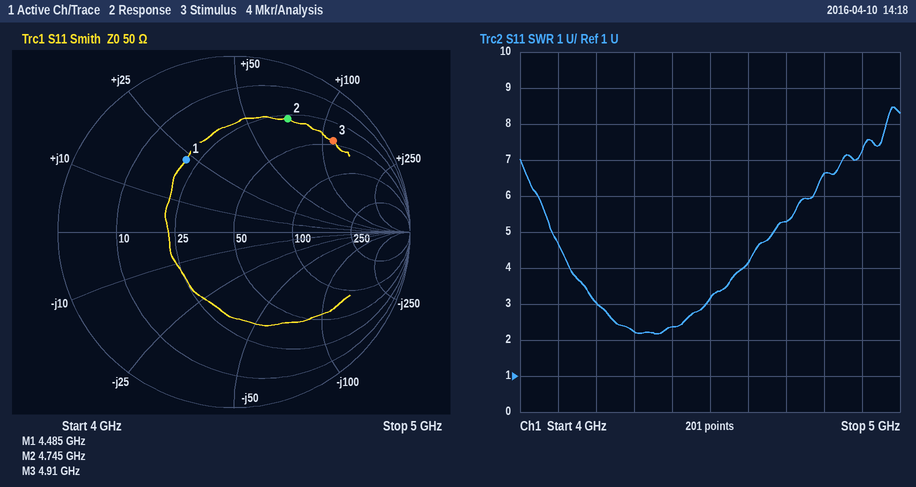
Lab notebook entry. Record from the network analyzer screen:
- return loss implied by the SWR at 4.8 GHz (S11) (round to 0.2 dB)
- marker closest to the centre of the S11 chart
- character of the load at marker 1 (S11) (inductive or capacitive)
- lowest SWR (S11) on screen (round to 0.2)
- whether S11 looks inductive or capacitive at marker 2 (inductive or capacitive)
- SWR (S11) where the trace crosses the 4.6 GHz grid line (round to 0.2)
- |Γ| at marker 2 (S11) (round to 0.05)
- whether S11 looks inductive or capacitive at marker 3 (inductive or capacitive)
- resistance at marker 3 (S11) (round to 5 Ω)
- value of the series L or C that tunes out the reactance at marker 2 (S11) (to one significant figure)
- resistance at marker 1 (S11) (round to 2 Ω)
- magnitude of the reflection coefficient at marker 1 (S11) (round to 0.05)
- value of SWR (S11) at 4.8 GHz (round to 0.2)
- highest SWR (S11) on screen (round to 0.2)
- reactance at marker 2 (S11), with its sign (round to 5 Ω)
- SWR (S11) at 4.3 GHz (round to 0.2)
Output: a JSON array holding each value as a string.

["2.6 dB", "marker 1", "inductive", "2.2", "inductive", "4.2", "0.70", "inductive", "45 Ω", "500 fF", "22 Ω", "0.50", "6.6", "8.4", "+70 Ω", "2.2"]
